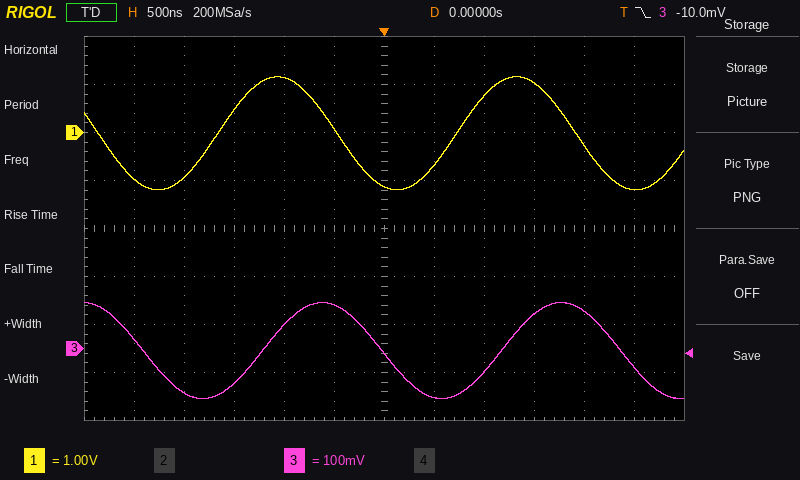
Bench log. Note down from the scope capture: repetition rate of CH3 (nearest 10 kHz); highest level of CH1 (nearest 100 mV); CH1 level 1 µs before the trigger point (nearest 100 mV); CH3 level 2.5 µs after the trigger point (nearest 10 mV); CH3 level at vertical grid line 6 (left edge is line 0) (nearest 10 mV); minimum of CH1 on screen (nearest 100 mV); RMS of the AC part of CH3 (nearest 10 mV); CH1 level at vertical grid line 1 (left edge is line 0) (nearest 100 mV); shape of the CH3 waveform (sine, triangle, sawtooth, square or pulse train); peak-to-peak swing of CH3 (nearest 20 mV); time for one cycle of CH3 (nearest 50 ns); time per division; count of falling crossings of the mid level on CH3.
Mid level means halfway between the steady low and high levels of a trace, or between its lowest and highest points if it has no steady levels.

420 kHz
1.2 V
1.1 V
-40 mV
-10 mV
-1.2 V
70 mV
-1.0 V
sine
200 mV
2.40 µs
500 ns
3
